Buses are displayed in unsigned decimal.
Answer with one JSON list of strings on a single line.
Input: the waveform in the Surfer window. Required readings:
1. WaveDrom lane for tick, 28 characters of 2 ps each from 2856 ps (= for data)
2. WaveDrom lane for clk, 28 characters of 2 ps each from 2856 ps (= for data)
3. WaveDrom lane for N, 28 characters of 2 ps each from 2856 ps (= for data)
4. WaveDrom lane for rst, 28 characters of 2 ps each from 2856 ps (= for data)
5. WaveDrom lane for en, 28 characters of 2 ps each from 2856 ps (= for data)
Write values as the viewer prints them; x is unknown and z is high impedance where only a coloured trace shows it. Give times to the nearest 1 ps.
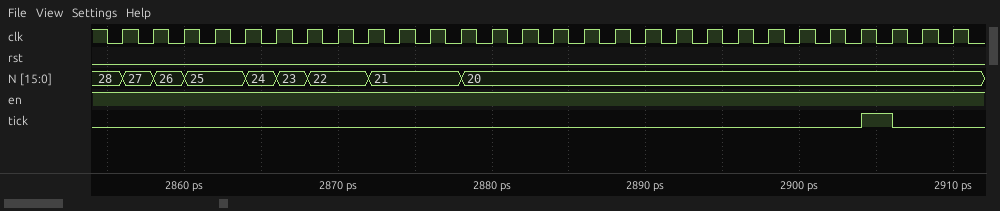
["{name: 'tick', wave: '0.......................10..'}", "{name: 'clk', wave: 'p...........................'}", "{name: 'N', wave: '===.===.=..=................', data: '27 26 25 24 23 22 21 20'}", "{name: 'rst', wave: '0...........................'}", "{name: 'en', wave: '1...........................'}"]
